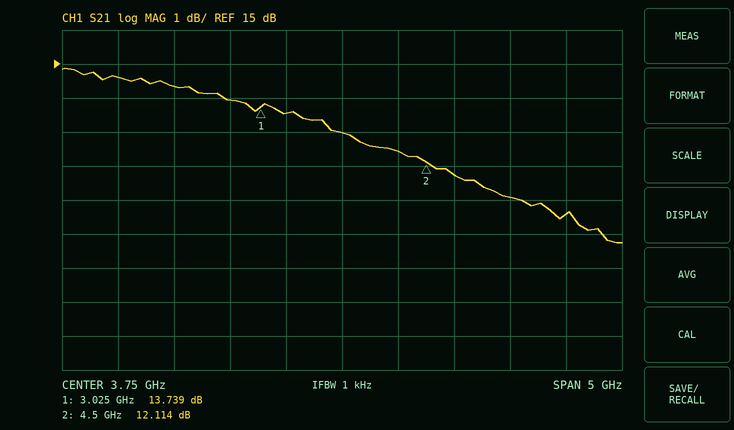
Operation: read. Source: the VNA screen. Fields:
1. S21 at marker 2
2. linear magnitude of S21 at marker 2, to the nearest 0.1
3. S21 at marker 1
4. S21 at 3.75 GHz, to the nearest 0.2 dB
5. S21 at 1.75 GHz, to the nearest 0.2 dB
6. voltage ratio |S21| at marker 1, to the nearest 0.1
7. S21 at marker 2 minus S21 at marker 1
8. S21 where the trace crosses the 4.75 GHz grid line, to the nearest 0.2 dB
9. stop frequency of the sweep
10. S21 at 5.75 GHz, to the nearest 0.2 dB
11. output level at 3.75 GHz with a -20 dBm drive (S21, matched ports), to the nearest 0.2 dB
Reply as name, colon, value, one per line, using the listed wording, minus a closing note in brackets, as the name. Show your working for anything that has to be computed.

S21 at marker 2: 12.114 dB
linear magnitude of S21 at marker 2, to the nearest 0.1: 10^(12.114/20) ≈ 4.0
S21 at marker 1: 13.739 dB
S21 at 3.75 GHz, to the nearest 0.2 dB: 13.0 dB
S21 at 1.75 GHz, to the nearest 0.2 dB: 14.6 dB
voltage ratio |S21| at marker 1, to the nearest 0.1: 10^(13.739/20) ≈ 4.9
S21 at marker 2 minus S21 at marker 1: 12.114 − (13.739) = -1.625 dB
S21 where the trace crosses the 4.75 GHz grid line, to the nearest 0.2 dB: 11.8 dB
stop frequency of the sweep: 6.25 GHz
S21 at 5.75 GHz, to the nearest 0.2 dB: 10.6 dB
output level at 3.75 GHz with a -20 dBm drive (S21, matched ports), to the nearest 0.2 dB: -20 dBm + (13.0 dB) = -7.0 dBm
